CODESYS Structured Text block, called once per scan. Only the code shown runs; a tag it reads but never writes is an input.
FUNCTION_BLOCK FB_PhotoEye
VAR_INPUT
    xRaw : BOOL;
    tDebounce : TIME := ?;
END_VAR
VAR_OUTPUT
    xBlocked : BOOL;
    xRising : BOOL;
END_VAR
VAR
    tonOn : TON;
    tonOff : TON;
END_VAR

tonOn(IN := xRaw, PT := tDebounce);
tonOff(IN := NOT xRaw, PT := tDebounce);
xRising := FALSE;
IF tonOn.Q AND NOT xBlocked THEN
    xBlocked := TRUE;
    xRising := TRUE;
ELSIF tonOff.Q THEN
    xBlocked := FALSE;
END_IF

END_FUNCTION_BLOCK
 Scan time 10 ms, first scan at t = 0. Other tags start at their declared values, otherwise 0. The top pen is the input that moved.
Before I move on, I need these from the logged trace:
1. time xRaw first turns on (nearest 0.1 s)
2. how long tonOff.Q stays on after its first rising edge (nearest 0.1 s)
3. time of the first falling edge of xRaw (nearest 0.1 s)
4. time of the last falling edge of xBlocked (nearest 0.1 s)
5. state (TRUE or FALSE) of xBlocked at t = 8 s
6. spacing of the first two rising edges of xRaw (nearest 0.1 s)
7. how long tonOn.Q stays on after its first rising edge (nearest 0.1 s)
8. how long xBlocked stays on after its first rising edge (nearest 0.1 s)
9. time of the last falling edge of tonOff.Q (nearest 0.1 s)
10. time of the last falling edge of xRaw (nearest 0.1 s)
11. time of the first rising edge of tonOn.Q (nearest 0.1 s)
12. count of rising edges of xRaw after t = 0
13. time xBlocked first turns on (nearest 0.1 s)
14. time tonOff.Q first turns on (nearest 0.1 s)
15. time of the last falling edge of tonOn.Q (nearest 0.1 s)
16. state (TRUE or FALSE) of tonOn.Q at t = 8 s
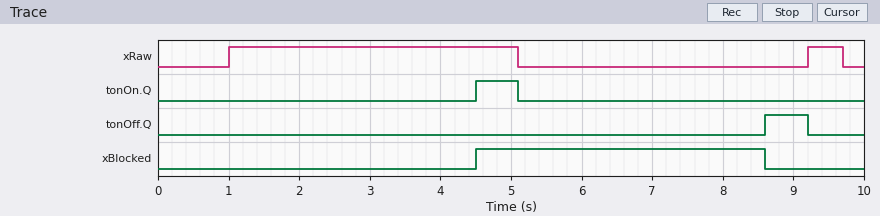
1.0 s
0.6 s
5.1 s
8.6 s
TRUE
8.2 s
0.6 s
4.1 s
9.2 s
9.7 s
4.5 s
2
4.5 s
8.6 s
5.1 s
FALSE
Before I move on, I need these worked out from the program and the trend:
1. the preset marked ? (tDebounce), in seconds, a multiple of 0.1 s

3.5 s
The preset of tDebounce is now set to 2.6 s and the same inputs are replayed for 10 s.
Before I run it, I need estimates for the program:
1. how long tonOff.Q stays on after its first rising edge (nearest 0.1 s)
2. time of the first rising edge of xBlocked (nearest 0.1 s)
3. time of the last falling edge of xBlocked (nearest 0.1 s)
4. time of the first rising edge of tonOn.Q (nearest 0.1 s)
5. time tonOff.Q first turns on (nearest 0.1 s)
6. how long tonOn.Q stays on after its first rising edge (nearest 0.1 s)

1.5 s
3.6 s
7.7 s
3.6 s
7.7 s
1.5 s
